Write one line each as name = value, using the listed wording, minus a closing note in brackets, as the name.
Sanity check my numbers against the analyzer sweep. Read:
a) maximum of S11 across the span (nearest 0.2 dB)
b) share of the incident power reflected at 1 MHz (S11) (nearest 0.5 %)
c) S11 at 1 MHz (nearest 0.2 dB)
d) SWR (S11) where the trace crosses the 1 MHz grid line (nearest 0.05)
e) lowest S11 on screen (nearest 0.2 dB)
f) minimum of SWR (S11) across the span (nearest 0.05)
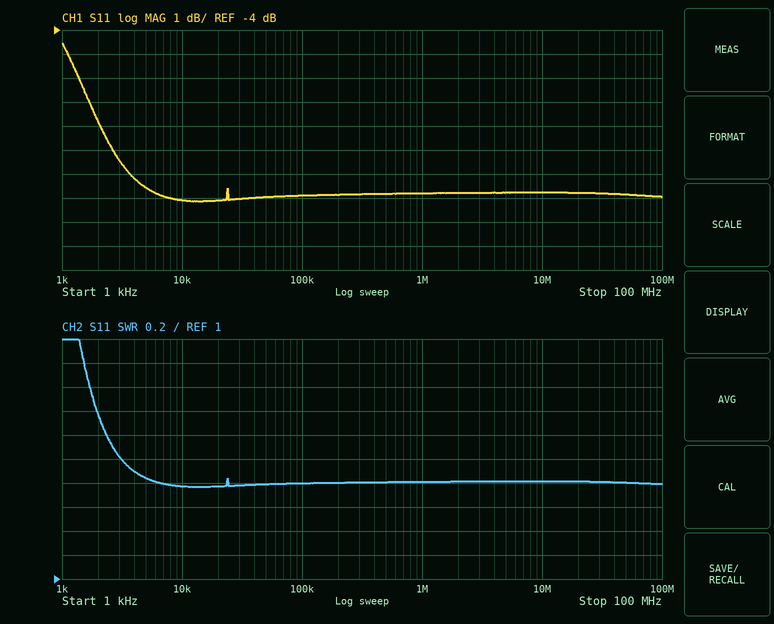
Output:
maximum of S11 across the span = -4.6 dB
share of the incident power reflected at 1 MHz (S11) = 8.5 %
S11 at 1 MHz = -10.8 dB
SWR (S11) where the trace crosses the 1 MHz grid line = 1.80
lowest S11 on screen = -11.2 dB
minimum of SWR (S11) across the span = 1.75
